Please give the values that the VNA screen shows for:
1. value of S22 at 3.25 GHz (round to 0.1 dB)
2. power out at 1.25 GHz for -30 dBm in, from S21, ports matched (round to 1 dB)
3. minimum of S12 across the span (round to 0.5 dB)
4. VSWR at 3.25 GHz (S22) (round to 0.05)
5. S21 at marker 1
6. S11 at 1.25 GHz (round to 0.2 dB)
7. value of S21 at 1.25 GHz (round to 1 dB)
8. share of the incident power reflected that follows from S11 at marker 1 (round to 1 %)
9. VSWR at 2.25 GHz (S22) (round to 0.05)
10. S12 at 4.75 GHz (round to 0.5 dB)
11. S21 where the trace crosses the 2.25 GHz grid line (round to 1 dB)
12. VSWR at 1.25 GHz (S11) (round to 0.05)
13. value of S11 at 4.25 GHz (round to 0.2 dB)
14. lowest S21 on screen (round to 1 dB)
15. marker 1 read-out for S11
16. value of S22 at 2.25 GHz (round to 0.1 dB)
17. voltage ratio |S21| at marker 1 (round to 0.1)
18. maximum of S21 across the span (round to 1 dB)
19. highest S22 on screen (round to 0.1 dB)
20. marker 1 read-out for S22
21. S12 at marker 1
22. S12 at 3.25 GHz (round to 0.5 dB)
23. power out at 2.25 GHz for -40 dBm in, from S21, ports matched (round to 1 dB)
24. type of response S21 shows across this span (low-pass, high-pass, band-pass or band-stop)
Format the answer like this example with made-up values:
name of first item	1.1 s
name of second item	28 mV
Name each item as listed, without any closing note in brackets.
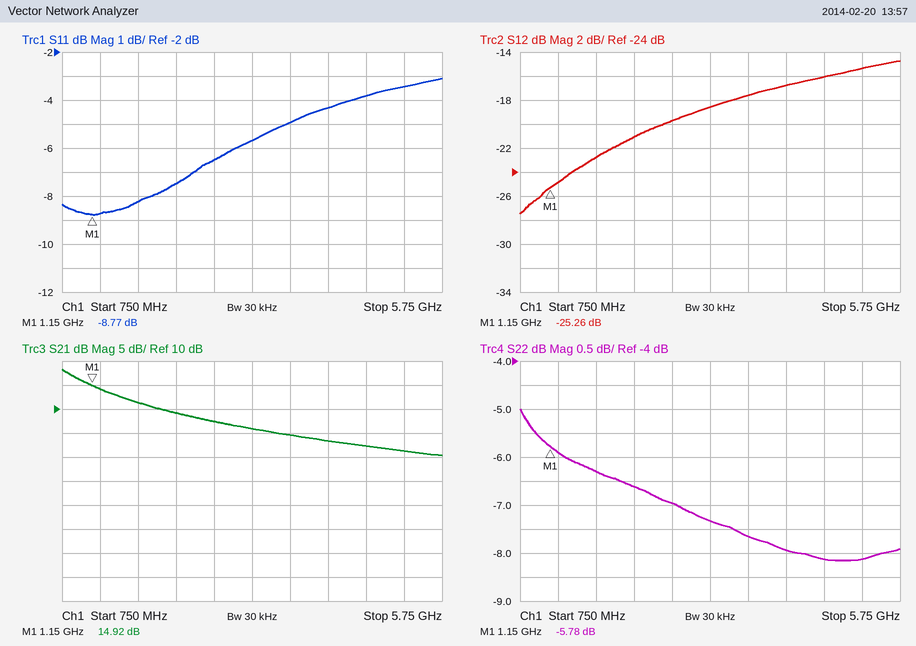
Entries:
value of S22 at 3.25 GHz	-7.3 dB
power out at 1.25 GHz for -30 dBm in, from S21, ports matched	-16 dBm
minimum of S12 across the span	-27.5 dB
VSWR at 3.25 GHz (S22)	2.50
S21 at marker 1	14.92 dB
S11 at 1.25 GHz	-8.8 dB
value of S21 at 1.25 GHz	14 dB
share of the incident power reflected that follows from S11 at marker 1	13 %
VSWR at 2.25 GHz (S22)	2.75
S12 at 4.75 GHz	-16.0 dB
S21 where the trace crosses the 2.25 GHz grid line	9 dB
VSWR at 1.25 GHz (S11)	2.15
value of S11 at 4.25 GHz	-4.4 dB
lowest S21 on screen	0 dB
marker 1 read-out for S11	-8.77 dB
value of S22 at 2.25 GHz	-6.6 dB
voltage ratio |S21| at marker 1	5.6
maximum of S21 across the span	18 dB
highest S22 on screen	-5.0 dB
marker 1 read-out for S22	-5.78 dB
S12 at marker 1	-25.26 dB
S12 at 3.25 GHz	-18.5 dB
power out at 2.25 GHz for -40 dBm in, from S21, ports matched	-31 dBm
type of response S21 shows across this span	low-pass
